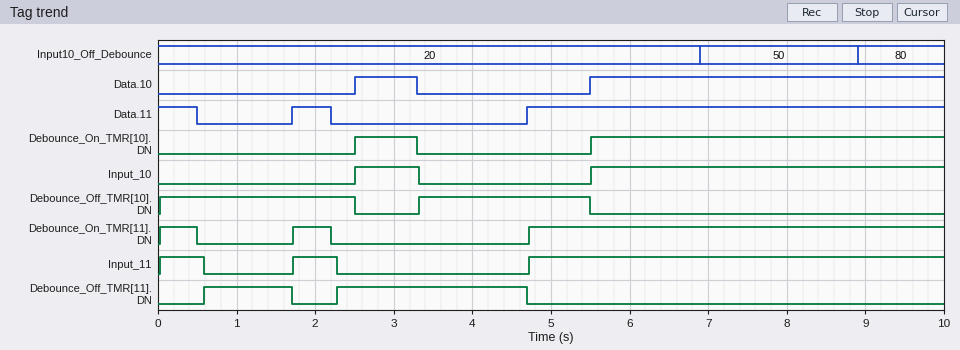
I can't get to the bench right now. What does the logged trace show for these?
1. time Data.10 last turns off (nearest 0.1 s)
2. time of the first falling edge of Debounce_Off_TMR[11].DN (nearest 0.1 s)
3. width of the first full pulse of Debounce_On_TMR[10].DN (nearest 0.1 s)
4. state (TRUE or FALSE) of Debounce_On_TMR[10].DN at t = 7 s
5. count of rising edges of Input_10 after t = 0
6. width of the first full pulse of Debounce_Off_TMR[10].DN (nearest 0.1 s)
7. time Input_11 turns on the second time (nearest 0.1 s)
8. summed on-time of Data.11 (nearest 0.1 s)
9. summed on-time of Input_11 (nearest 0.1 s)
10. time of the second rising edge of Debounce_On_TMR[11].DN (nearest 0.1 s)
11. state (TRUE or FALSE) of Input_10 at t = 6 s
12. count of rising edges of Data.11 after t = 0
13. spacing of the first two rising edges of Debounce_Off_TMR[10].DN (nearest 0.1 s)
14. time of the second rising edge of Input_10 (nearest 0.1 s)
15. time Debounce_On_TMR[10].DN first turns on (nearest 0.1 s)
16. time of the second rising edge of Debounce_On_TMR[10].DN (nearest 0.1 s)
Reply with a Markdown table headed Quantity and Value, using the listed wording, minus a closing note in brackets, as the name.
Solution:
| Quantity | Value |
|---|---|
| time Data.10 last turns off | 3.3 s |
| time of the first falling edge of Debounce_Off_TMR[11].DN | 1.7 s |
| width of the first full pulse of Debounce_On_TMR[10].DN | 0.8 s |
| state (TRUE or FALSE) of Debounce_On_TMR[10].DN at t = 7 s | TRUE |
| count of rising edges of Input_10 after t = 0 | 2 |
| width of the first full pulse of Debounce_Off_TMR[10].DN | 2.5 s |
| time Input_11 turns on the second time | 1.7 s |
| summed on-time of Data.11 | 6.3 s |
| summed on-time of Input_11 | 6.4 s |
| time of the second rising edge of Debounce_On_TMR[11].DN | 1.7 s |
| state (TRUE or FALSE) of Input_10 at t = 6 s | TRUE |
| count of rising edges of Data.11 after t = 0 | 2 |
| spacing of the first two rising edges of Debounce_Off_TMR[10].DN | 3.3 s |
| time of the second rising edge of Input_10 | 5.5 s |
| time Debounce_On_TMR[10].DN first turns on | 2.5 s |
| time of the second rising edge of Debounce_On_TMR[10].DN | 5.5 s |
